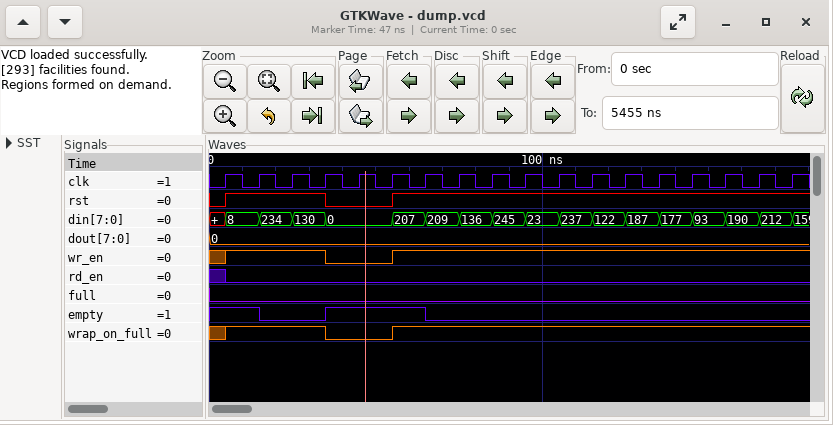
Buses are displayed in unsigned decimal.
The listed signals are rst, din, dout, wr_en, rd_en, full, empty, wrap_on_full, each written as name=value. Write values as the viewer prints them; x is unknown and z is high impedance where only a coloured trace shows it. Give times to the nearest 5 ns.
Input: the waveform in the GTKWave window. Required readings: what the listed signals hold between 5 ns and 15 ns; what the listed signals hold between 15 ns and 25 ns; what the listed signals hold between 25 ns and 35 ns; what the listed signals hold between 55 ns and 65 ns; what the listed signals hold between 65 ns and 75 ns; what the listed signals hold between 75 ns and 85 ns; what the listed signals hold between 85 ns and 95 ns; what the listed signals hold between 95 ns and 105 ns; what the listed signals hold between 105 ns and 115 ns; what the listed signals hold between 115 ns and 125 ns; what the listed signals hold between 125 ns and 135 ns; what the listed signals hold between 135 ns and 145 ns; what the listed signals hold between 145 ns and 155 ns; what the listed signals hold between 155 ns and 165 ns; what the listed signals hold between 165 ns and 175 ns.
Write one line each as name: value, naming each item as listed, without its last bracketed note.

what the listed signals hold between 5 ns and 15 ns: rst=1, din=8, dout=0, wr_en=1, rd_en=0, full=0, empty=1, wrap_on_full=1
what the listed signals hold between 15 ns and 25 ns: rst=1, din=234, dout=0, wr_en=1, rd_en=0, full=0, empty=0, wrap_on_full=1
what the listed signals hold between 25 ns and 35 ns: rst=1, din=130, dout=0, wr_en=1, rd_en=0, full=0, empty=0, wrap_on_full=1
what the listed signals hold between 55 ns and 65 ns: rst=1, din=207, dout=0, wr_en=1, rd_en=0, full=0, empty=1, wrap_on_full=1
what the listed signals hold between 65 ns and 75 ns: rst=1, din=209, dout=0, wr_en=1, rd_en=0, full=0, empty=0, wrap_on_full=1
what the listed signals hold between 75 ns and 85 ns: rst=1, din=136, dout=0, wr_en=1, rd_en=0, full=0, empty=0, wrap_on_full=1
what the listed signals hold between 85 ns and 95 ns: rst=1, din=245, dout=0, wr_en=1, rd_en=0, full=0, empty=0, wrap_on_full=1
what the listed signals hold between 95 ns and 105 ns: rst=1, din=23, dout=0, wr_en=1, rd_en=0, full=0, empty=0, wrap_on_full=1
what the listed signals hold between 105 ns and 115 ns: rst=1, din=237, dout=0, wr_en=1, rd_en=0, full=0, empty=0, wrap_on_full=1
what the listed signals hold between 115 ns and 125 ns: rst=1, din=122, dout=0, wr_en=1, rd_en=0, full=0, empty=0, wrap_on_full=1
what the listed signals hold between 125 ns and 135 ns: rst=1, din=187, dout=0, wr_en=1, rd_en=0, full=0, empty=0, wrap_on_full=1
what the listed signals hold between 135 ns and 145 ns: rst=1, din=177, dout=0, wr_en=1, rd_en=0, full=0, empty=0, wrap_on_full=1
what the listed signals hold between 145 ns and 155 ns: rst=1, din=93, dout=0, wr_en=1, rd_en=0, full=0, empty=0, wrap_on_full=1
what the listed signals hold between 155 ns and 165 ns: rst=1, din=190, dout=0, wr_en=1, rd_en=0, full=0, empty=0, wrap_on_full=1
what the listed signals hold between 165 ns and 175 ns: rst=1, din=212, dout=0, wr_en=1, rd_en=0, full=0, empty=0, wrap_on_full=1
